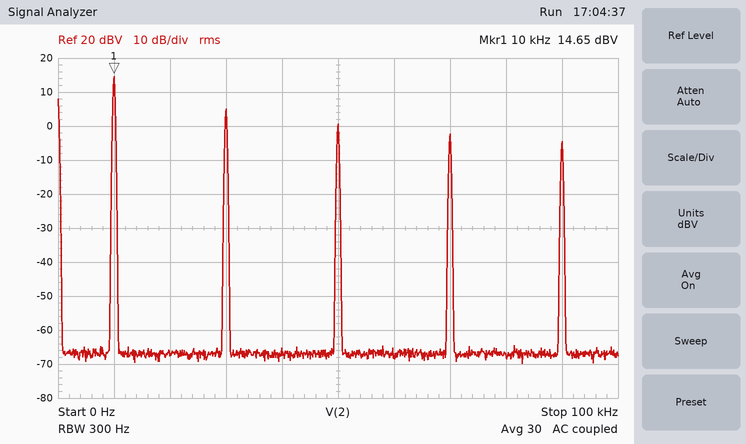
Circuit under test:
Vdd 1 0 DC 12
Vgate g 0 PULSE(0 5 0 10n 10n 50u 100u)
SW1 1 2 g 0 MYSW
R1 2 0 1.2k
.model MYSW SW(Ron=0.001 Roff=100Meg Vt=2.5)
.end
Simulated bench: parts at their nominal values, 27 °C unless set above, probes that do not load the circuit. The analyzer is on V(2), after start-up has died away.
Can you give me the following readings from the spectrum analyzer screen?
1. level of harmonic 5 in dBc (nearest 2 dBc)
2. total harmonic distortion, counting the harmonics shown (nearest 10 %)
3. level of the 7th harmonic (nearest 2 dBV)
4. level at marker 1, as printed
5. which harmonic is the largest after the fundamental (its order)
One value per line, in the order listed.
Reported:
-14 dBc
40 %
-2 dBV
14.65 dBV
3
